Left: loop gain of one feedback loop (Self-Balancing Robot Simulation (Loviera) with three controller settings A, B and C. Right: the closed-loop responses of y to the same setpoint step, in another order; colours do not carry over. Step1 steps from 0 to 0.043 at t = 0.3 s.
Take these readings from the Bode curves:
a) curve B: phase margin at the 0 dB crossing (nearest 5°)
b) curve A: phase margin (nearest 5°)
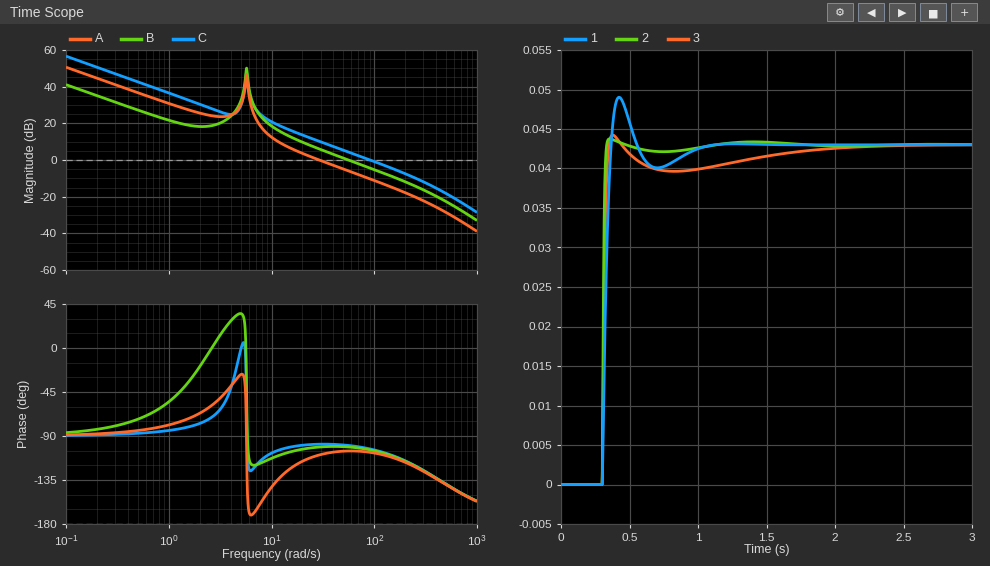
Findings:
80°
70°
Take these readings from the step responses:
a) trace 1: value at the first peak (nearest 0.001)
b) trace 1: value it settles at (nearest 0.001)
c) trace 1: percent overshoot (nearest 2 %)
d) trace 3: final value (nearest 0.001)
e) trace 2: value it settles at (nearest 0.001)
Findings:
0.049
0.043
14 %
0.043
0.043
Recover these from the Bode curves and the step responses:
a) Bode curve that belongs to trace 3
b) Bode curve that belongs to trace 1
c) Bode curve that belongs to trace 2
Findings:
B
A
C
